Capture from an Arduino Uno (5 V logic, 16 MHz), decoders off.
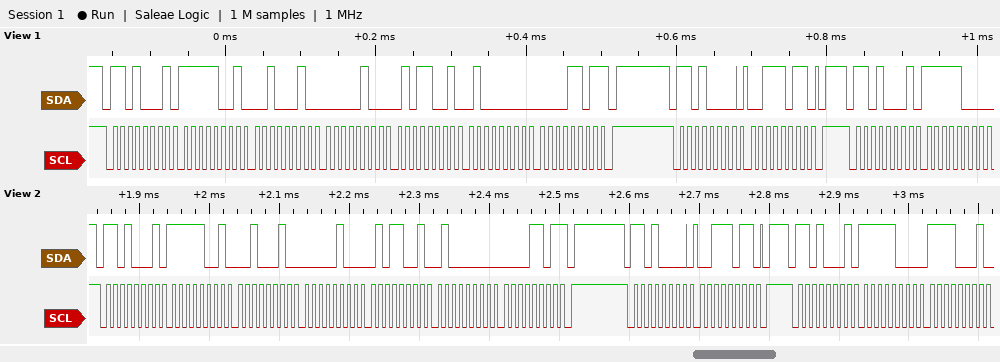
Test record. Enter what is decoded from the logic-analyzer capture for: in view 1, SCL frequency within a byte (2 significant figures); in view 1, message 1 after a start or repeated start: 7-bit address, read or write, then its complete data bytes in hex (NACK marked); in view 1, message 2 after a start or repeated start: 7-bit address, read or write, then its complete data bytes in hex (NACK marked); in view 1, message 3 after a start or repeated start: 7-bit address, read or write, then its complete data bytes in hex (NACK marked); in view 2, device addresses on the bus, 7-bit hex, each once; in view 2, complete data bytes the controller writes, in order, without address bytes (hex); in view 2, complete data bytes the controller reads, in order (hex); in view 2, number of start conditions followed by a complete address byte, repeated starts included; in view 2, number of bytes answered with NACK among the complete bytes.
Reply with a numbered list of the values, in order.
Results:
1. 100 kHz
2. 0x68 read: F9 22 04 59 40 0D NACK
3. 0x68 write: 3B
4. 0x68 read: F8
5. 0x68
6. 3B
7. F9 22 04 59 40 0D F8 F1
8. 3
9. 1
